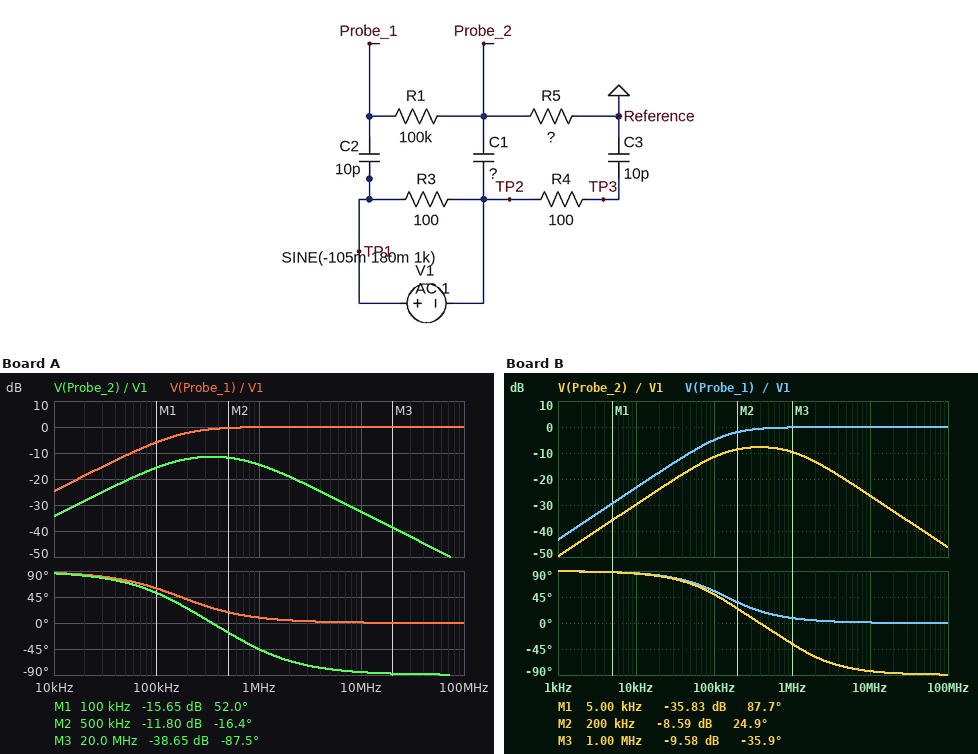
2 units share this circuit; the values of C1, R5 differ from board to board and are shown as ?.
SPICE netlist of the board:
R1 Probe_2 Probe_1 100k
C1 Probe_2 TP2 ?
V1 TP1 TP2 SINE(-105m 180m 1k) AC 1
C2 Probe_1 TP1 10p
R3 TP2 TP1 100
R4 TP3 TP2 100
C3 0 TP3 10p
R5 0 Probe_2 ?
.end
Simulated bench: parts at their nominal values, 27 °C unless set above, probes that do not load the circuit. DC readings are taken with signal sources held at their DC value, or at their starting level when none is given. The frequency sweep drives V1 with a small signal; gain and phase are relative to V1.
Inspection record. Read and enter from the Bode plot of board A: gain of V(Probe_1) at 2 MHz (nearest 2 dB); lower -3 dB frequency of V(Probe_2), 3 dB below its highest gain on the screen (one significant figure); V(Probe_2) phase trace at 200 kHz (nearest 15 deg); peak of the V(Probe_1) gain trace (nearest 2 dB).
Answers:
0 dB
100 kHz
30 deg
0 dB
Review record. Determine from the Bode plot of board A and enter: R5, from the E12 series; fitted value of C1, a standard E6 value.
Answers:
82 kΩ
6.8 pF
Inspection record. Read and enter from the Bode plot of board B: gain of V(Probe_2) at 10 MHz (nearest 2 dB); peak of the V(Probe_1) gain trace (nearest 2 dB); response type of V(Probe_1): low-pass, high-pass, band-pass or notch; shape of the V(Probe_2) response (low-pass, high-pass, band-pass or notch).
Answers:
-26 dB
0 dB
high-pass
band-pass
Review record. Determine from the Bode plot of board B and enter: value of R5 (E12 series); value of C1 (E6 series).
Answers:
120 kΩ
3.3 pF
